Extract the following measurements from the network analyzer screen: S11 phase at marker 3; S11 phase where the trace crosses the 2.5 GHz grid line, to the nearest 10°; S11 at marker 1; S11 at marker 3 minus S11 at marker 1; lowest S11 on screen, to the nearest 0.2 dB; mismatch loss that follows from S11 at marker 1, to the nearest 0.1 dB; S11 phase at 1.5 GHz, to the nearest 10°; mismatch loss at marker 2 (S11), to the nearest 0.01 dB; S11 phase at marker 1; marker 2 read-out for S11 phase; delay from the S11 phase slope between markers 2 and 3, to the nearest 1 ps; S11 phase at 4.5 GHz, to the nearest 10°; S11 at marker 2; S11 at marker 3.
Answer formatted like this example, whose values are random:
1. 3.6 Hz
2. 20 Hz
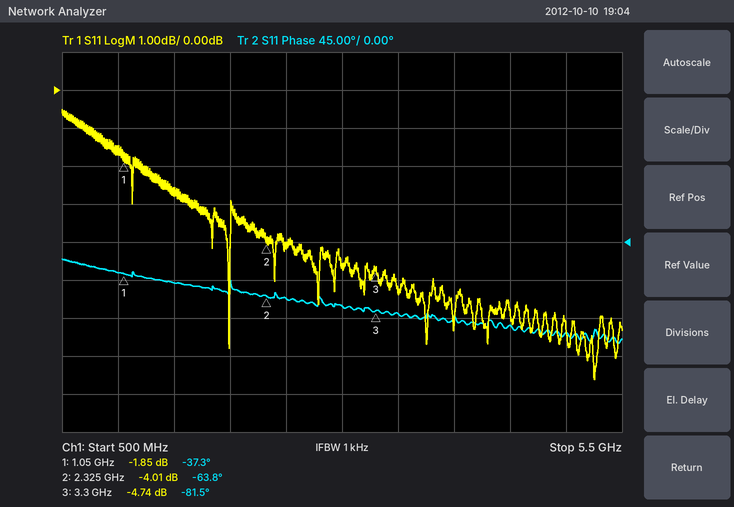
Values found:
1. -81.5°
2. -70°
3. -1.85 dB
4. -2.89 dB
5. -7.6 dB
6. 4.6 dB
7. -50°
8. 2.20 dB
9. -37.3°
10. -63.8°
11. 50 ps
12. -100°
13. -4.01 dB
14. -4.74 dB
